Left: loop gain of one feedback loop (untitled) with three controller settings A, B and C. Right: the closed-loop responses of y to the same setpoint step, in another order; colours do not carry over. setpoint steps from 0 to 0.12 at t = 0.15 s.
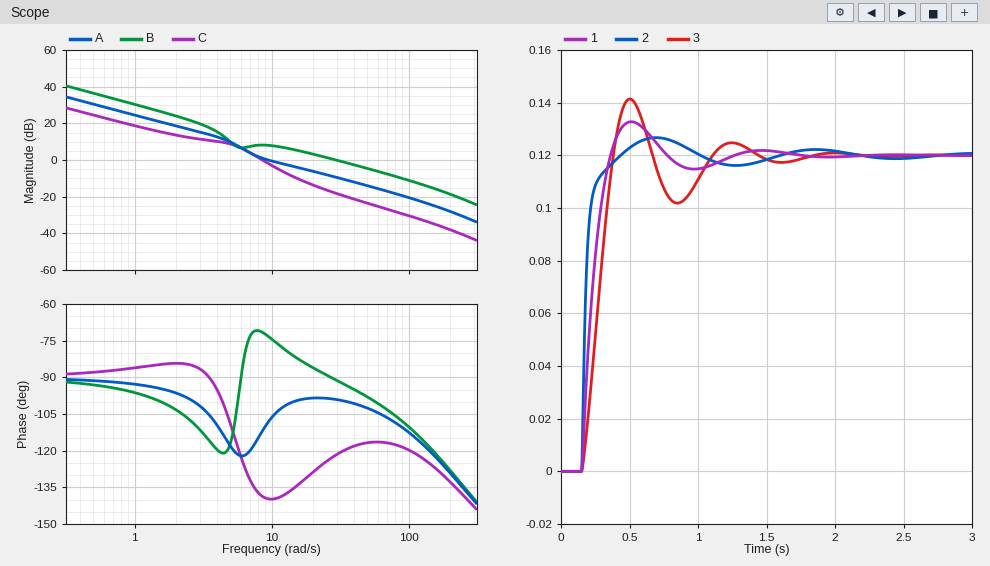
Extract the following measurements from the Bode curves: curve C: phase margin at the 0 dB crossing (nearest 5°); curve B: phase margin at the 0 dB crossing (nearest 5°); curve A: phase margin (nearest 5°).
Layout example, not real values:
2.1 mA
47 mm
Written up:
40°
90°
70°
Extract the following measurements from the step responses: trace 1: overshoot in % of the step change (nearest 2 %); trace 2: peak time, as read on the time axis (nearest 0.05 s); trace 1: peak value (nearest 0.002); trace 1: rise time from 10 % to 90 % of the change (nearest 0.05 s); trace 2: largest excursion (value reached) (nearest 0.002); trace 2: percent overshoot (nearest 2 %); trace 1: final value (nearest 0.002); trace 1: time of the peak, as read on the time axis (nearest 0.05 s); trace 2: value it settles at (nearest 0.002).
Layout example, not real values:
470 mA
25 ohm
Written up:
10 %
0.70 s
0.132
0.15 s
0.126
6 %
0.120
0.50 s
0.120
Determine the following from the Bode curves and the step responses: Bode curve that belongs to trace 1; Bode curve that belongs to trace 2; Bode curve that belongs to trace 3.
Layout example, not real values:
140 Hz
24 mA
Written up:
A
B
C
